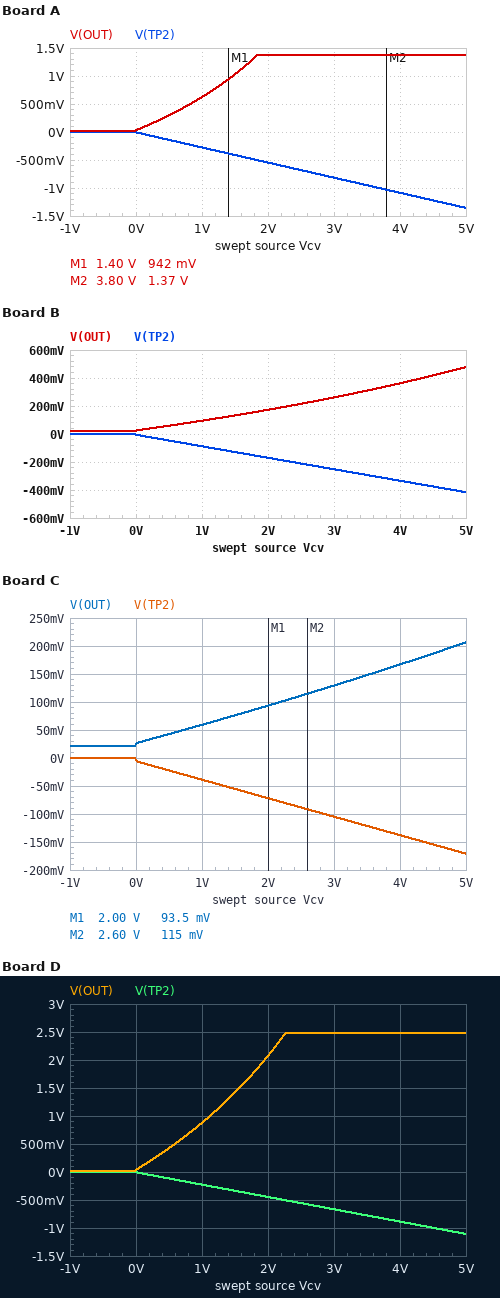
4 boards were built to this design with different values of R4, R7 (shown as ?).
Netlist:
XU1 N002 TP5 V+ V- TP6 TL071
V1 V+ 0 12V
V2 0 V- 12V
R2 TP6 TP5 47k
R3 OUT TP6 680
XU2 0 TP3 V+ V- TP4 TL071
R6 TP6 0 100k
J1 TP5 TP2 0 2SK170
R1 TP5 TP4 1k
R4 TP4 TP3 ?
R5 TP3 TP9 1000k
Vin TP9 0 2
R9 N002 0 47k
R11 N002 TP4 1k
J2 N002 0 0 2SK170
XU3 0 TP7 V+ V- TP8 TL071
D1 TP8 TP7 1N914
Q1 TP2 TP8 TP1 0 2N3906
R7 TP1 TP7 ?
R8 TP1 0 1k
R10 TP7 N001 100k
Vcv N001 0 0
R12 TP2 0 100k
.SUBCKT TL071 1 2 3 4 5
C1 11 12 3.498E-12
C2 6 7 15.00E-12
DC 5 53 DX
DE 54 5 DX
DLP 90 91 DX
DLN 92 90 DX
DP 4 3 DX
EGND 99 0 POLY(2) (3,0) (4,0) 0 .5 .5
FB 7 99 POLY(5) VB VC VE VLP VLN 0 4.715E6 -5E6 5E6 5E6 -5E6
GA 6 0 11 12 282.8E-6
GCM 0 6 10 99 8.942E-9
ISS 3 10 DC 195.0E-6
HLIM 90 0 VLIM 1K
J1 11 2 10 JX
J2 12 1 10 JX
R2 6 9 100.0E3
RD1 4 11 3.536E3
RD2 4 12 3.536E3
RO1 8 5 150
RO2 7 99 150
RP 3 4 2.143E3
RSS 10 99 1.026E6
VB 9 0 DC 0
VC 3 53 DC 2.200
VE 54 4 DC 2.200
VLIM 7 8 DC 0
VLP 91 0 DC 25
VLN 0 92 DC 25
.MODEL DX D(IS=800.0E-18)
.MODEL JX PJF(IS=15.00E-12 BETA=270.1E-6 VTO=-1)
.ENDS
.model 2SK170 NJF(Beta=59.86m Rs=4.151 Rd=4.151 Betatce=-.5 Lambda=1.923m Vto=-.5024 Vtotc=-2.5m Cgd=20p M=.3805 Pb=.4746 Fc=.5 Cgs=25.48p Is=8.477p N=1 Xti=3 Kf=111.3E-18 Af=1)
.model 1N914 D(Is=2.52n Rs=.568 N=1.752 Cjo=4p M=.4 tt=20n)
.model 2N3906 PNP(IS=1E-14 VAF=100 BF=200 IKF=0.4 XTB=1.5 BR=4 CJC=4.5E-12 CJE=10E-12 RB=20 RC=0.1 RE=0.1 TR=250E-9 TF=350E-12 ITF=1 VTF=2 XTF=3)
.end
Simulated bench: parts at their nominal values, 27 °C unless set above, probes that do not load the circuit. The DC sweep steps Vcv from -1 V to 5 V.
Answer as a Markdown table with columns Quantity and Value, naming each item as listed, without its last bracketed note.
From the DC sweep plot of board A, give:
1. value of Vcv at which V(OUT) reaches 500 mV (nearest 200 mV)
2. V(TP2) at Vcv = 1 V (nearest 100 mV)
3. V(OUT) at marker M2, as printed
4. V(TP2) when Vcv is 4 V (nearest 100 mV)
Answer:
| Quantity | Value |
|---|---|
| value of Vcv at which V(OUT) reaches 500 mV | 800 mV |
| V(TP2) at Vcv = 1 V | -300 mV |
| V(OUT) at marker M2, as printed | 1.37 V |
| V(TP2) when Vcv is 4 V | -1.1 V |
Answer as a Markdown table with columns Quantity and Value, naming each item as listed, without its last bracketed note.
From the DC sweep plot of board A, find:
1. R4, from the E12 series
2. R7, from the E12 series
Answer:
| Quantity | Value |
|---|---|
| R4, from the E12 series | 15 kΩ |
| R7, from the E12 series | 27 kΩ |
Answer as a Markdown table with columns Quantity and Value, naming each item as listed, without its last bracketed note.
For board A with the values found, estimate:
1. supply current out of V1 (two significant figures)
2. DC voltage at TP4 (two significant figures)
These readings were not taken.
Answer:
| Quantity | Value |
|---|---|
| supply current out of V1 | 34 mA |
| DC voltage at TP4 | -30 mV |
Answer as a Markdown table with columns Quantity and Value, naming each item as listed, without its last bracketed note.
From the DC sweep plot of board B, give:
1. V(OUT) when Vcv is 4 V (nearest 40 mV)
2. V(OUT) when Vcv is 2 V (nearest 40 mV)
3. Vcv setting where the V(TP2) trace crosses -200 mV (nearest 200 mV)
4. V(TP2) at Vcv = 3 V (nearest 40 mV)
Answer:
| Quantity | Value |
|---|---|
| V(OUT) when Vcv is 4 V | 360 mV |
| V(OUT) when Vcv is 2 V | 160 mV |
| Vcv setting where the V(TP2) trace crosses -200 mV | 2.4 V |
| V(TP2) at Vcv = 3 V | -240 mV |
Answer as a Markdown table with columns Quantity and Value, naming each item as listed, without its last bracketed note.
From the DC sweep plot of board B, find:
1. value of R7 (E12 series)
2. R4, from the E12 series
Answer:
| Quantity | Value |
|---|---|
| value of R7 | 8.2 kΩ |
| R4, from the E12 series | 6.8 kΩ |
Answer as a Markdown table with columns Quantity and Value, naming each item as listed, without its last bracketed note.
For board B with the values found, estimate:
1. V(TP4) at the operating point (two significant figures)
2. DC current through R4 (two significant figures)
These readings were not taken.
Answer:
| Quantity | Value |
|---|---|
| V(TP4) at the operating point | -14 mV |
| DC current through R4 | 2.0 µA |
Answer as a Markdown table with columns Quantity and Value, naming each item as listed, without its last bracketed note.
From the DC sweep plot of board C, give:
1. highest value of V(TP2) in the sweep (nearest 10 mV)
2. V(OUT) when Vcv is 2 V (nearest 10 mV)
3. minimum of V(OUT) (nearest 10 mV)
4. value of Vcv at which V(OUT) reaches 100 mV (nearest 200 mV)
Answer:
| Quantity | Value |
|---|---|
| highest value of V(TP2) in the sweep | 0 V |
| V(OUT) when Vcv is 2 V | 90 mV |
| minimum of V(OUT) | 20 mV |
| value of Vcv at which V(OUT) reaches 100 mV | 2.2 V |
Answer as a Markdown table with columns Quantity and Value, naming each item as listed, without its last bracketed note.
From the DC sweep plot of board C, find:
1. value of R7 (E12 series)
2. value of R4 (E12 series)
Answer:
| Quantity | Value |
|---|---|
| value of R7 | 3.3 kΩ |
| value of R4 | 8.2 kΩ |
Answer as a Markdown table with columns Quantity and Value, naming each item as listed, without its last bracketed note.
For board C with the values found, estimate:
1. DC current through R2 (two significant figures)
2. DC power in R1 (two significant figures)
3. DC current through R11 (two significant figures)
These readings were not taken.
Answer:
| Quantity | Value |
|---|---|
| DC current through R2 | 460 nA |
| DC power in R1 | 260 nW |
| DC current through R11 | 16 µA |
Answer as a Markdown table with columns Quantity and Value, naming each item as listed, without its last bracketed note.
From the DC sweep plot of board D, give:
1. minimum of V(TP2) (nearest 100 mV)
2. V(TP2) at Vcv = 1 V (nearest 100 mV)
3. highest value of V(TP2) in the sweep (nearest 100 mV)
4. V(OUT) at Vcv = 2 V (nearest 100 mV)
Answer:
| Quantity | Value |
|---|---|
| minimum of V(TP2) | -1.1 V |
| V(TP2) at Vcv = 1 V | -200 mV |
| highest value of V(TP2) in the sweep | 0 V |
| V(OUT) at Vcv = 2 V | 2.1 V |
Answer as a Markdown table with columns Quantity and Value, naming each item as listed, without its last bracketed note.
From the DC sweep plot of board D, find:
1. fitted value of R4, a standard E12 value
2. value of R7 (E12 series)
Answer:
| Quantity | Value |
|---|---|
| fitted value of R4, a standard E12 value | 27 kΩ |
| value of R7 | 22 kΩ |
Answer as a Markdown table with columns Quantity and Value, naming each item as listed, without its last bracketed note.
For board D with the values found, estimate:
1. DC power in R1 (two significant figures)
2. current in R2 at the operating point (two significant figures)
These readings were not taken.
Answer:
| Quantity | Value |
|---|---|
| DC power in R1 | 2.8 µW |
| current in R2 at the operating point | 480 nA |
